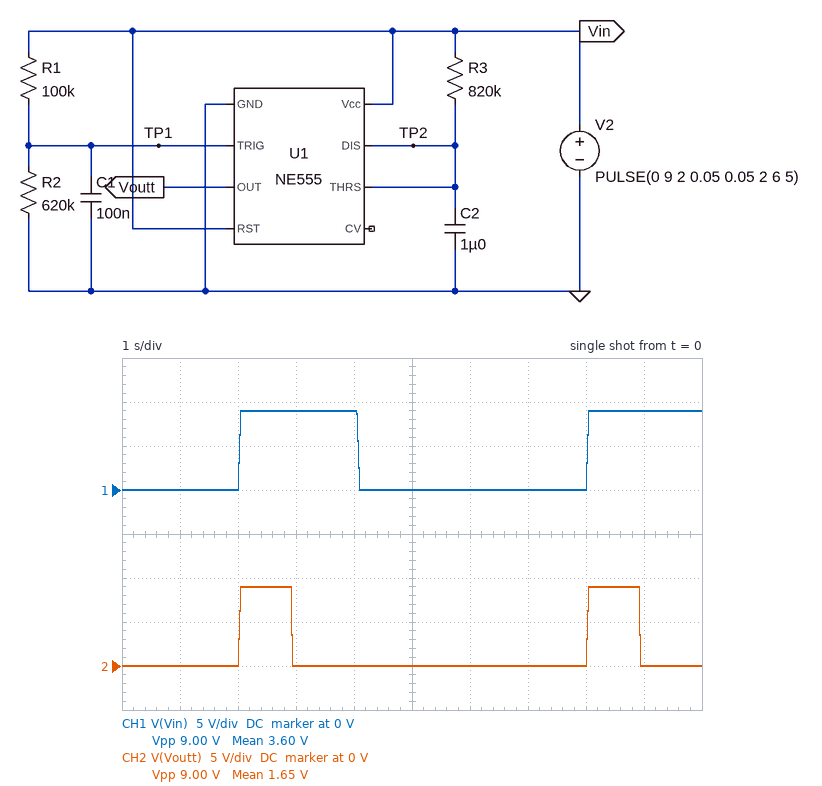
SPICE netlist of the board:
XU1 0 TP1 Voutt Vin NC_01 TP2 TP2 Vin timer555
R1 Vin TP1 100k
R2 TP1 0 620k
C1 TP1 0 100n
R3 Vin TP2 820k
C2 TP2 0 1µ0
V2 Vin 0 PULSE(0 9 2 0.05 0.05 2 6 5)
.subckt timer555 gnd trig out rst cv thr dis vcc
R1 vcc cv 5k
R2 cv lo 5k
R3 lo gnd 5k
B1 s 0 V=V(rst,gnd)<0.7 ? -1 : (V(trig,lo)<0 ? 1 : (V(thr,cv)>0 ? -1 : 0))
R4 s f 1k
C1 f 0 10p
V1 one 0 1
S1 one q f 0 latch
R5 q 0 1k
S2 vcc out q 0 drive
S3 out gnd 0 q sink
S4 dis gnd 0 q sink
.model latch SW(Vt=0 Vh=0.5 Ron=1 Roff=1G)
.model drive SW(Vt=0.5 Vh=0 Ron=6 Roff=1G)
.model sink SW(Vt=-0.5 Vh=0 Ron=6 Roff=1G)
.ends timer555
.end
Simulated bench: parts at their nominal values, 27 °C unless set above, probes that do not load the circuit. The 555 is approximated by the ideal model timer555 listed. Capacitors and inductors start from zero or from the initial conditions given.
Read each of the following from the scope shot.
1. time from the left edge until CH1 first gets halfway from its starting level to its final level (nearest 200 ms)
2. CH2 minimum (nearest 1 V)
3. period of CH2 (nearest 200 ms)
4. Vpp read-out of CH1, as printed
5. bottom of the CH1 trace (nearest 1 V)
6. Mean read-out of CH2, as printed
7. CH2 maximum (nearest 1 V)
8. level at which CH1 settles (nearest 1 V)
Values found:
2.0 s
0 V
6.0 s
9.00 V
0 V
1.65 V
9 V
9 V
